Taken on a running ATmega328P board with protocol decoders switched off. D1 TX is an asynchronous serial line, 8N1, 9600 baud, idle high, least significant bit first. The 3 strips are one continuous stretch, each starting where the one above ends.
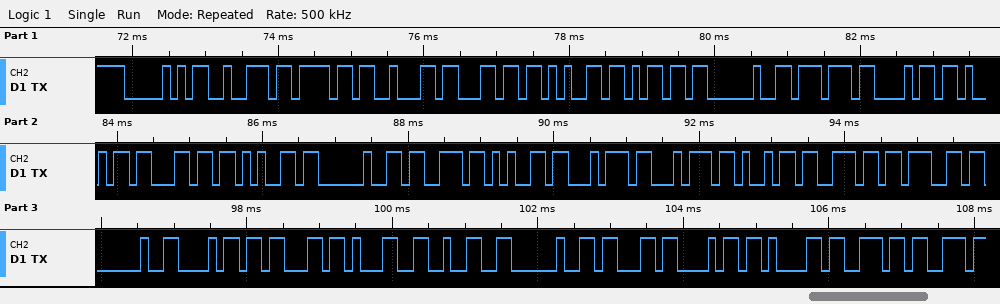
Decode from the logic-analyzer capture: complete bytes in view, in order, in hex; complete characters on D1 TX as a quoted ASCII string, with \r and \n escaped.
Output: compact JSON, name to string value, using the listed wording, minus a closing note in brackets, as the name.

{"complete bytes in view, in order, in hex": "50 72 6F 62 6C 65 6D 20 77 68 69 6C 65 20 73 65 74 74 69 6E 67 20 68 63 31 32 20 63 68 61 6E", "complete characters on D1 TX as a quoted ASCII string, with \\r and \\n escaped": "\"Problem while setting hc12 chan\""}
